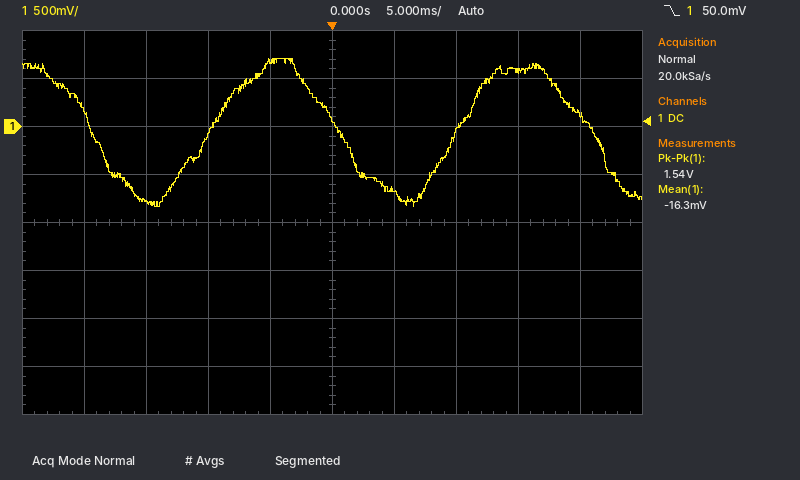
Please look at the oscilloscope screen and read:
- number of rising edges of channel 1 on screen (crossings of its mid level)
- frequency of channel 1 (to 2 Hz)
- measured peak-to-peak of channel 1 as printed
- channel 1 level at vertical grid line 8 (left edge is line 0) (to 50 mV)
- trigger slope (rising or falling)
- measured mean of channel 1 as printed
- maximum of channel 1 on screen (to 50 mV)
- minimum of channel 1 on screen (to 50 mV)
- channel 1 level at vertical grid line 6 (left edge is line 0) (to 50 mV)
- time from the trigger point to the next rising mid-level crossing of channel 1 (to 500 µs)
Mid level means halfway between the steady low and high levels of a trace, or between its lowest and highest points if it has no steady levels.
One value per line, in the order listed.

2
50 Hz
1.54 V
600 mV
falling
-16.3 mV
700 mV
-850 mV
-650 mV
10.0 ms
